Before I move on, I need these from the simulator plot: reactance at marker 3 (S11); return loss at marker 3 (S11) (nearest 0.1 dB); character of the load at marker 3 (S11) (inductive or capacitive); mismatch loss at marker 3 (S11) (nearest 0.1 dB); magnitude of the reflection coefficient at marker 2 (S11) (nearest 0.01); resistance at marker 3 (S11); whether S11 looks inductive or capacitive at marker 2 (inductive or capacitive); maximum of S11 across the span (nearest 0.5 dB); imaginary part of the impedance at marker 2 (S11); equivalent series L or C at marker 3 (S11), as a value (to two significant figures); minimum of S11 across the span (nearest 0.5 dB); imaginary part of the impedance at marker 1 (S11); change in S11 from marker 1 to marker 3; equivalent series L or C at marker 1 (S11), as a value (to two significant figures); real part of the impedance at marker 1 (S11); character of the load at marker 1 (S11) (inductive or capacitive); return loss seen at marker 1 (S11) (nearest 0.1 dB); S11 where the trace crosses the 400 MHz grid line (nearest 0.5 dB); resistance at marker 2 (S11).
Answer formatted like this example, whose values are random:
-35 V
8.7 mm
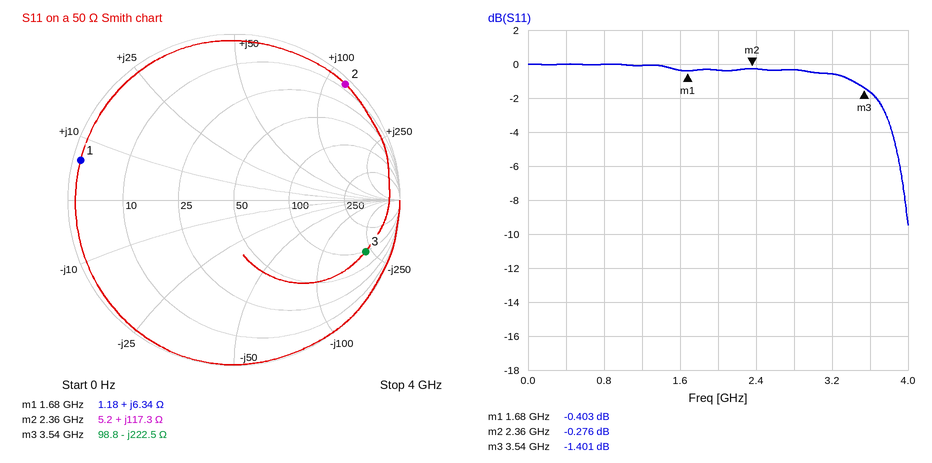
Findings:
-222.5 Ω
1.4 dB
capacitive
5.6 dB
0.97
98.8 Ω
inductive
0.0 dB
+117.3 Ω
200 fF
-9.5 dB
+6.34 Ω
-0.998 dB
600 pH
1.18 Ω
inductive
0.4 dB
0.0 dB
5.2 Ω
